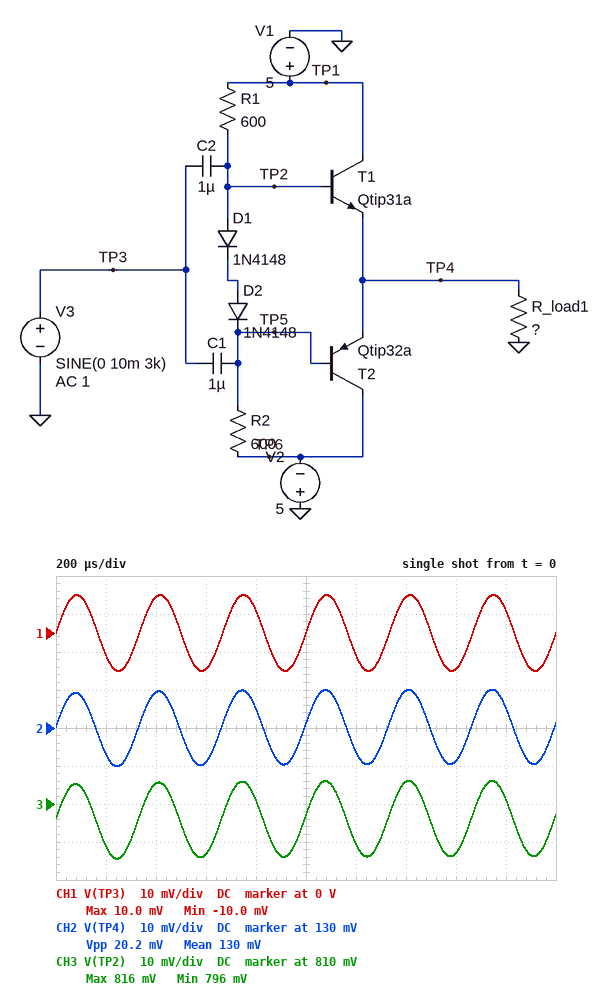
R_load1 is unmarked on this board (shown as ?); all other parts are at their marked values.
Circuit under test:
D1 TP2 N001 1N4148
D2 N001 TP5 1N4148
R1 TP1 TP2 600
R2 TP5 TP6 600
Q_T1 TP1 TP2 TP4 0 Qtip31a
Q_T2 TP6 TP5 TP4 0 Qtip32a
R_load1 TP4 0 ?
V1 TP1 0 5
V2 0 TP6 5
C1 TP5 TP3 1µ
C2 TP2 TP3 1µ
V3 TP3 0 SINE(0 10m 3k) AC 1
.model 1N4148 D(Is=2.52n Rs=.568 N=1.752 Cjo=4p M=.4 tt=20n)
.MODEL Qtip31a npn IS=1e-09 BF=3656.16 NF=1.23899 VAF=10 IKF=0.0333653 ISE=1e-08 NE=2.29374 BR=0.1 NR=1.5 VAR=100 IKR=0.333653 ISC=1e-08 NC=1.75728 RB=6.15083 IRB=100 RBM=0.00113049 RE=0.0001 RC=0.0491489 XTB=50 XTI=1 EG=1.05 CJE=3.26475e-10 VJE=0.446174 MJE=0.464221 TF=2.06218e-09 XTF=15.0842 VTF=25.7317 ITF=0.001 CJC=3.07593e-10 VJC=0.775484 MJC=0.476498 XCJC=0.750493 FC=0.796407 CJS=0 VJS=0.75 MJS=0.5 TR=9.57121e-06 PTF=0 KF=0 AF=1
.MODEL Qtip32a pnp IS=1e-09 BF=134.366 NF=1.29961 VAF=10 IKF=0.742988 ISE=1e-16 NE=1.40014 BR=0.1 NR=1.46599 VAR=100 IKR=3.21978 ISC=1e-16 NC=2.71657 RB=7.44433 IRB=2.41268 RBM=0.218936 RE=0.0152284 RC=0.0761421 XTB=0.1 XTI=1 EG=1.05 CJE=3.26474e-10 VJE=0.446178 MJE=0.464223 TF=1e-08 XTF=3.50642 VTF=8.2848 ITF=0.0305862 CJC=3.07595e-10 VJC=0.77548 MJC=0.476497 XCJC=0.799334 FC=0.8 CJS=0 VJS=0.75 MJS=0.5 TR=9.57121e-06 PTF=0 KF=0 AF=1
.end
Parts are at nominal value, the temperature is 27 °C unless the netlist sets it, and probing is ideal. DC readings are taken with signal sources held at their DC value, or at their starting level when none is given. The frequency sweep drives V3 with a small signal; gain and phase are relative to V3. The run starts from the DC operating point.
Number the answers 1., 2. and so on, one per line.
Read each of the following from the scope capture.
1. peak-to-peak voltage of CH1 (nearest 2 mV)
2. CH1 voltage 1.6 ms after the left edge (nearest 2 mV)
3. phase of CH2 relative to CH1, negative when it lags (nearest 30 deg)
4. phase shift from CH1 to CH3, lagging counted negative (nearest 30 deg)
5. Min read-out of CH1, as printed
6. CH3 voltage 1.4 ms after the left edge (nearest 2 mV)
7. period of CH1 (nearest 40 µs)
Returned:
1. 20 mV
2. -10 mV
3. 0 deg
4. 0 deg
5. -10.0 mV
6. 816 mV
7. 320 µs
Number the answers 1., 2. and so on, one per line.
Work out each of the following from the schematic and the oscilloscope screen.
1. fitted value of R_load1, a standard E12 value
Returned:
1. 15 Ω
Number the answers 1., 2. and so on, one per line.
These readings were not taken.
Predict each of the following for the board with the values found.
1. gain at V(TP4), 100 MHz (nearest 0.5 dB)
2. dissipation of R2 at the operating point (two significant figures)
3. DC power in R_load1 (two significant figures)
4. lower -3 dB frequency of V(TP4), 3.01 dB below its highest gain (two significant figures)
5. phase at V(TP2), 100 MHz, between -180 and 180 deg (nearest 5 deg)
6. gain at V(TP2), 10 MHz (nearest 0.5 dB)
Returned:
1. -2.5 dB
2. 33 mW
3. 1.1 mW
4. 320 Hz
5. 0 deg
6. 0 dB
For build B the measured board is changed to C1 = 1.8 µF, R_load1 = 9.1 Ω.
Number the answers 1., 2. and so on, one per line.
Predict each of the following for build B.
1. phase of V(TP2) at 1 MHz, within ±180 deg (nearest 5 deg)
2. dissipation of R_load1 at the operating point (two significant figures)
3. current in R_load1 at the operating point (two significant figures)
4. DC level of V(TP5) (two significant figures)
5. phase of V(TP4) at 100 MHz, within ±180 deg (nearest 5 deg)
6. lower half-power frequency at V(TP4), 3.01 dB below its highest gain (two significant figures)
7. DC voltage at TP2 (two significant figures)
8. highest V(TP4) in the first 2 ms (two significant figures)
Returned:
1. 0 deg
2. 1.6 mW
3. 13 mA
4. -540 mV
5. -15 deg
6. 240 Hz
7. 800 mV
8. 130 mV
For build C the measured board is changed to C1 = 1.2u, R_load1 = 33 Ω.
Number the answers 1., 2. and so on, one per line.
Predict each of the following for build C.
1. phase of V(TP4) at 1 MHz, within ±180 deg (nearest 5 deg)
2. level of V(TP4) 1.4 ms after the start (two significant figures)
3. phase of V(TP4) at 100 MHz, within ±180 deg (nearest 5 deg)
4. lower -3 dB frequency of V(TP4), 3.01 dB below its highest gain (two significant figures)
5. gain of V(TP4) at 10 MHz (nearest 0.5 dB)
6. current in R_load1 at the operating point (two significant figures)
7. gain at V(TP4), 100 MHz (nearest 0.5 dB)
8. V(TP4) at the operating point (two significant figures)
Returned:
1. 0 deg
2. 150 mV
3. -20 deg
4. 270 Hz
5. -1.0 dB
6. 4.2 mA
7. -2.0 dB
8. 140 mV
